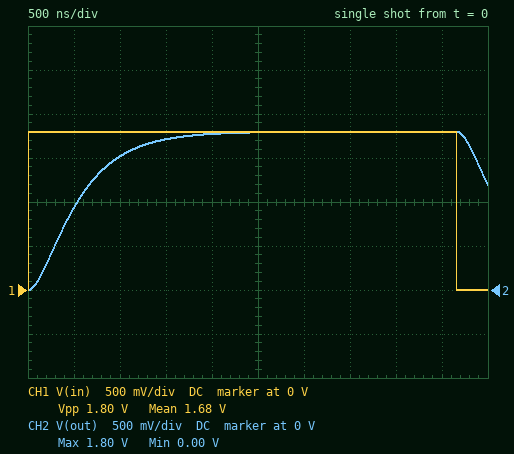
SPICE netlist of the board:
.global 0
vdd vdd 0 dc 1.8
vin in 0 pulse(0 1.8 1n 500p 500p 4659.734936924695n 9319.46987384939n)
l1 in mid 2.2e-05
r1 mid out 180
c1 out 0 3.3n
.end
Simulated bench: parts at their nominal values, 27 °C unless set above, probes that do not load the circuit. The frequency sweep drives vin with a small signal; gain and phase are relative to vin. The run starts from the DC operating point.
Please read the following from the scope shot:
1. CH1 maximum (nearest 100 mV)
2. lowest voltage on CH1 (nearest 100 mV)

1.8 V
0 V
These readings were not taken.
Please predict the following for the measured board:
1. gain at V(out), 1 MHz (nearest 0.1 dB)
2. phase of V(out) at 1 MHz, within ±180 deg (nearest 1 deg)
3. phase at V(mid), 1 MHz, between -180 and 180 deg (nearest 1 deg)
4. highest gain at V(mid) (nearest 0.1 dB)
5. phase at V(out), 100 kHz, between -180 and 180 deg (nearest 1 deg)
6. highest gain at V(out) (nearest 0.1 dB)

-12.4 dB
-117 deg
-42 deg
1.1 dB
-21 deg
0 dB
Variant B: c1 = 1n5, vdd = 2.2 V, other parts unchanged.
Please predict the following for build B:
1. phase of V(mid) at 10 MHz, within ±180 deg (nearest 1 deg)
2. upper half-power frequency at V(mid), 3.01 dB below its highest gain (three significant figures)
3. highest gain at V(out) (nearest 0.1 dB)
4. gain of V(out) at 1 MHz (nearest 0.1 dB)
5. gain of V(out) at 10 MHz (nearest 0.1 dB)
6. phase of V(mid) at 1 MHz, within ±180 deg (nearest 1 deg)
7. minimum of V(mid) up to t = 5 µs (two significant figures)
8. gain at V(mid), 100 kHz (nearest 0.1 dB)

-86 deg
1.44 MHz
0 dB
-4.7 dB
-42.3 dB
-41 deg
-330 mV
0.1 dB
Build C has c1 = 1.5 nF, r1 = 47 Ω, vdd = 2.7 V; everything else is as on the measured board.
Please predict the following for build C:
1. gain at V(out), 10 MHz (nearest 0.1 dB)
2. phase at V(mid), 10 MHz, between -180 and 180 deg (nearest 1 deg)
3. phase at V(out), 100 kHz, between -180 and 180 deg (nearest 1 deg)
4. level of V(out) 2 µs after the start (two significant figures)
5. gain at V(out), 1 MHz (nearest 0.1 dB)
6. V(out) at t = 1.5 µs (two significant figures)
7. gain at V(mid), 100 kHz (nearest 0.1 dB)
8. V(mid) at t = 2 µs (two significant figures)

-42.2 dB
-101 deg
-3 deg
1.9 V
5.4 dB
1.8 V
0.1 dB
1.8 V
